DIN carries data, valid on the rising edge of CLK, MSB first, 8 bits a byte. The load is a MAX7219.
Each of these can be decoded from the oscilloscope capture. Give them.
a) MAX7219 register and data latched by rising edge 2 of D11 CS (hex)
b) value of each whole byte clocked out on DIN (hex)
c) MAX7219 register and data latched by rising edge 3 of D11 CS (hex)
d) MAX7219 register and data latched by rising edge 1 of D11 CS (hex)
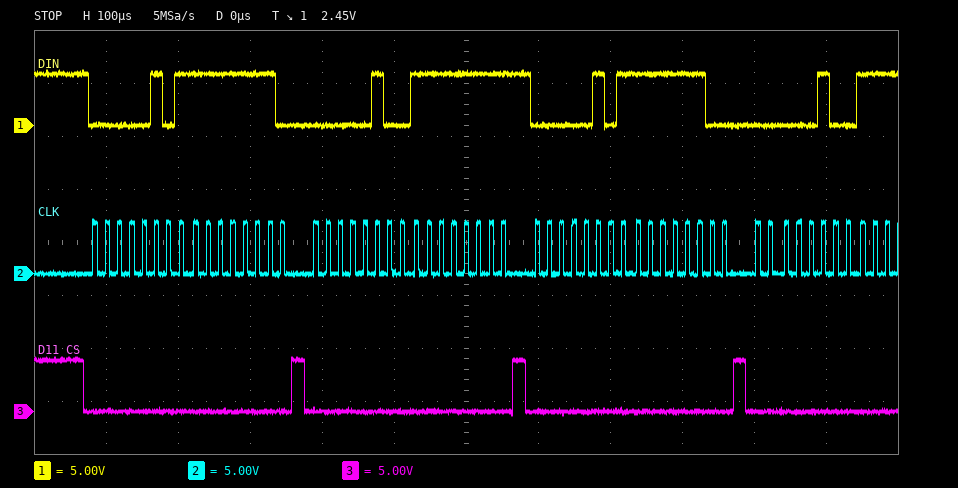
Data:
register 0x4, data 0xFF
0x05 0xFE 0x04 0xFF 0x05 0xFC 0x04
register 0x5, data 0xFC
register 0x5, data 0xFE
